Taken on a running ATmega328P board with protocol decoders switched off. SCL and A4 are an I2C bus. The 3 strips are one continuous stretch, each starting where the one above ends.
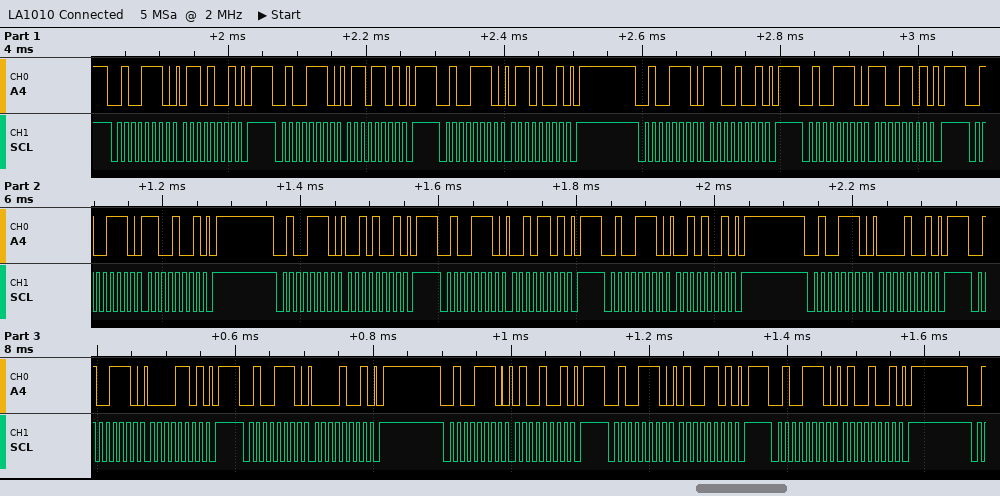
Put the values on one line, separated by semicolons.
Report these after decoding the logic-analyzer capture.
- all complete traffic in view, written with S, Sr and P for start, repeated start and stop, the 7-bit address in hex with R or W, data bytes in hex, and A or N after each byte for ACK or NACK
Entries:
S 27W A 69 A P S 27W A 6D A P S 27W A 69 A P S 27W A C9 A P S 27W A CD A P S 27W A C9 A P S 27W A 29 A P S 27W A 2D A P S 27W A 29 A P S 27W A 09 A P S 27W A 0D A P S 27W A 09 A P S 27W A 49 A P S 27W A 4D A P S 27W A 49 A P
